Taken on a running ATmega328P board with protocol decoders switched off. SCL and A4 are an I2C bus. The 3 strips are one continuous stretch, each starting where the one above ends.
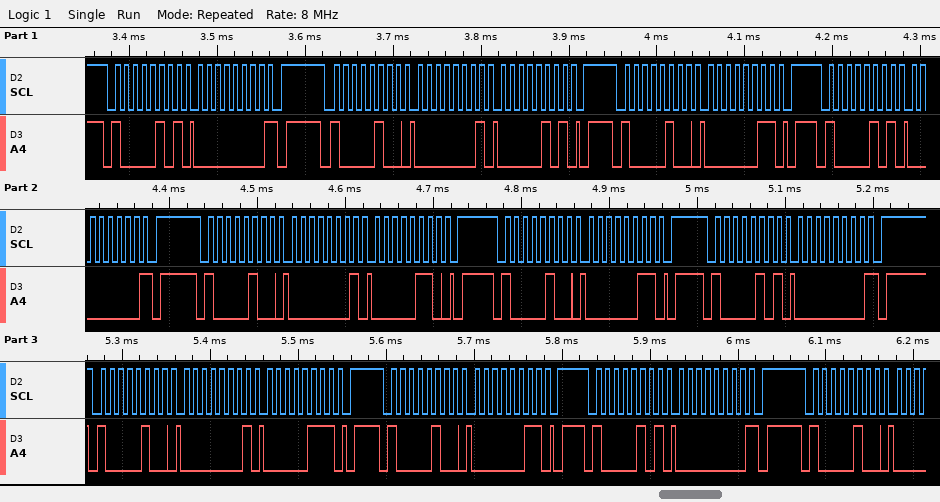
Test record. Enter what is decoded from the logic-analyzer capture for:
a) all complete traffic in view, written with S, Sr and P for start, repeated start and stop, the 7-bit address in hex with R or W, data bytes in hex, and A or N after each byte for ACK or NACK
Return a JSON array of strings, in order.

["S 42R A 00 N P S 42W A 01 A 05 A P S 42W A 03 A P S 42R A 00 N P S 42W A 01 A 06 A P S 42W A 03 A P S 42R A 00 N P S 42W A 01 A 07 A P S 42W A 03 A P S 42R A 00 N P S 42W A"]
